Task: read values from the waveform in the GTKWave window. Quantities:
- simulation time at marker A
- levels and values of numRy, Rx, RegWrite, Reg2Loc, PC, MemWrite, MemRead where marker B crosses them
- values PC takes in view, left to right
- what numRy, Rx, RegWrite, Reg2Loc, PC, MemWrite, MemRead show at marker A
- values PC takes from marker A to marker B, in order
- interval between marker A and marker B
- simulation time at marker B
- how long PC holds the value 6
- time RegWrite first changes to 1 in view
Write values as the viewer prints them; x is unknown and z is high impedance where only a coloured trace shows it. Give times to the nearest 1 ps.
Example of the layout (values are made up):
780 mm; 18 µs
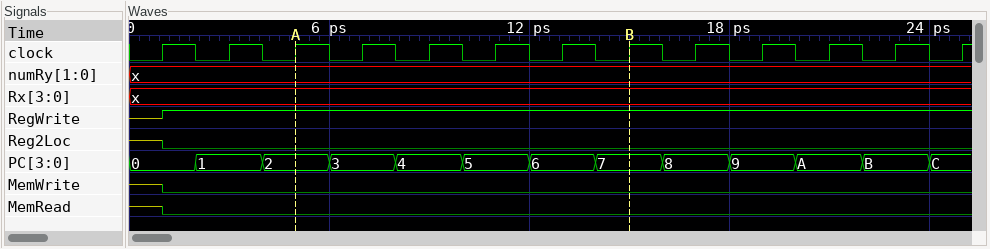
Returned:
5 ps; numRy=x, Rx=x, RegWrite=1, Reg2Loc=0, PC=7, MemWrite=0, MemRead=0; 0, 1, 2, 3, 4, 5, 6, 7, 8, 9, A, B, C; numRy=x, Rx=x, RegWrite=1, Reg2Loc=0, PC=2, MemWrite=0, MemRead=0; 2, 3, 4, 5, 6, 7; 10 ps; 15 ps; 2 ps; 1 ps
